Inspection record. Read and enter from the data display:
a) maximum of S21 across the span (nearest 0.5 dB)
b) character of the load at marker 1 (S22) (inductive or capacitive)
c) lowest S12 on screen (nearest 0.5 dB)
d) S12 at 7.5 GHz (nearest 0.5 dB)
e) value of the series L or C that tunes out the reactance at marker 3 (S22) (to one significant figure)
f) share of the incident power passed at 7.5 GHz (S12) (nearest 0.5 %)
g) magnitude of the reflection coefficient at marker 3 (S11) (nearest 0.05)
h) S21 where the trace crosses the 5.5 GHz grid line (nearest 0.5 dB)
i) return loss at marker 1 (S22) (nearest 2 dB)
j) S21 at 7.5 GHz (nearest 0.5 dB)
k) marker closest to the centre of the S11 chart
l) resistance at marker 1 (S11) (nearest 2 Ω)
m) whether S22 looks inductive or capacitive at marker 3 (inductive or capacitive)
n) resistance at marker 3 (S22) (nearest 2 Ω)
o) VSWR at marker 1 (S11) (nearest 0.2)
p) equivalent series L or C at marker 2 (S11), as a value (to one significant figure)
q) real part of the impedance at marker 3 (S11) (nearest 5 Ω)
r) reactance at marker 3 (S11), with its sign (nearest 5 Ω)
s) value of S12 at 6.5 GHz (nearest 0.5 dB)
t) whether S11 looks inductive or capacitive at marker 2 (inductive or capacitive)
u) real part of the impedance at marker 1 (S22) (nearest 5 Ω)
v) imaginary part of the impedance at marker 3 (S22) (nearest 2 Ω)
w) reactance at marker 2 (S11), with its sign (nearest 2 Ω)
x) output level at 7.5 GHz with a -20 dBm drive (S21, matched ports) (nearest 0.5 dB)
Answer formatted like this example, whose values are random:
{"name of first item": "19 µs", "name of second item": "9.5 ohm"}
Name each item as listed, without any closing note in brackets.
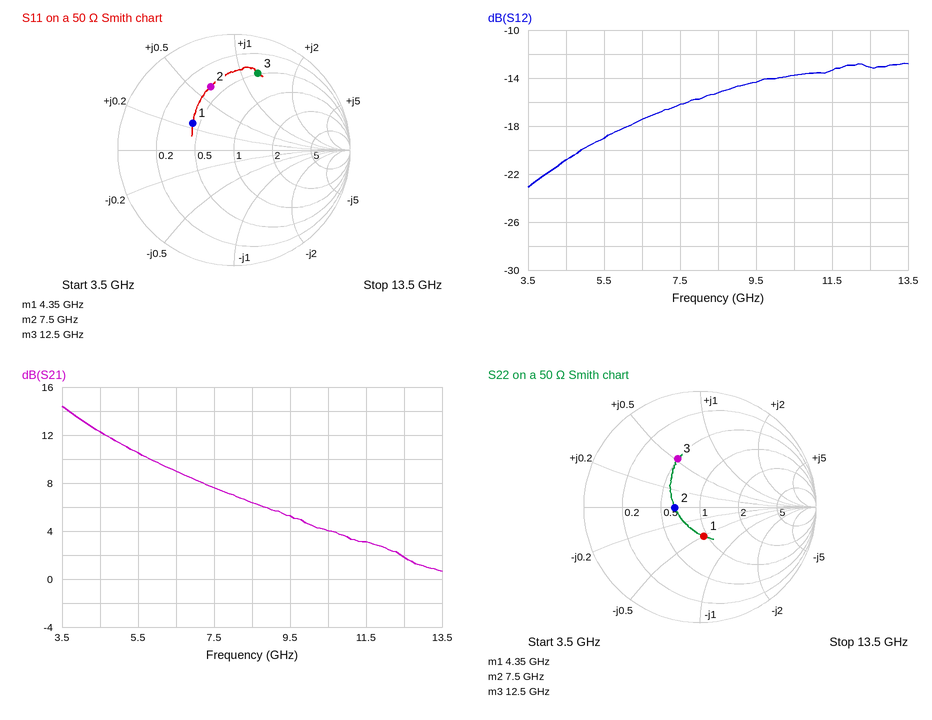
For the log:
{"maximum of S21 across the span": "14.5 dB", "character of the load at marker 1 (S22)": "capacitive", "lowest S12 on screen": "-23.0 dB", "S12 at 7.5 GHz": "-16.0 dB", "value of the series L or C that tunes out the reactance at marker 3 (S22)": "500 fF", "share of the incident power passed at 7.5 GHz (S12)": "2.5 %", "magnitude of the reflection coefficient at marker 3 (S11)": "0.70", "S21 where the trace crosses the 5.5 GHz grid line": "10.5 dB", "return loss at marker 1 (S22)": "12 dB", "S21 at 7.5 GHz": "7.5 dB", "marker closest to the centre of the S11 chart": "marker 1", "resistance at marker 1 (S11)": "22 Ω", "whether S22 looks inductive or capacitive at marker 3": "inductive", "resistance at marker 3 (S22)": "24 Ω", "VSWR at marker 1 (S11)": "2.4", "equivalent series L or C at marker 2 (S11), as a value": "700 pH", "real part of the impedance at marker 3 (S11)": "25 Ω", "reactance at marker 3 (S11), with its sign": "+60 Ω", "value of S12 at 6.5 GHz": "-17.5 dB", "whether S11 looks inductive or capacitive at marker 2": "inductive", "real part of the impedance at marker 1 (S22)": "45 Ω", "imaginary part of the impedance at marker 3 (S22)": "+26 Ω", "reactance at marker 2 (S11), with its sign": "+32 Ω", "output level at 7.5 GHz with a -20 dBm drive (S21, matched ports)": "-12.5 dBm"}
